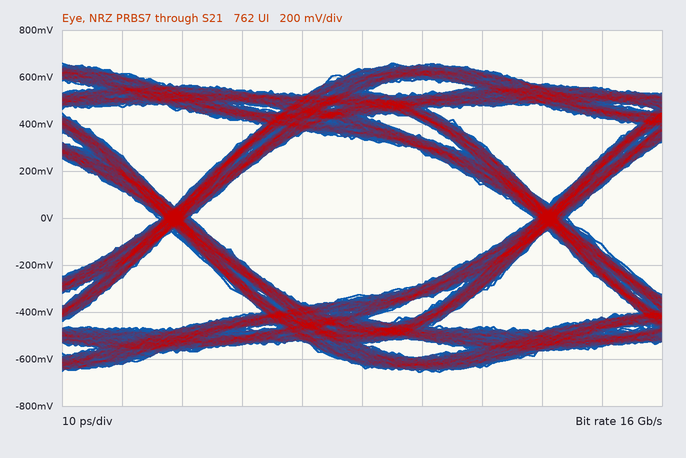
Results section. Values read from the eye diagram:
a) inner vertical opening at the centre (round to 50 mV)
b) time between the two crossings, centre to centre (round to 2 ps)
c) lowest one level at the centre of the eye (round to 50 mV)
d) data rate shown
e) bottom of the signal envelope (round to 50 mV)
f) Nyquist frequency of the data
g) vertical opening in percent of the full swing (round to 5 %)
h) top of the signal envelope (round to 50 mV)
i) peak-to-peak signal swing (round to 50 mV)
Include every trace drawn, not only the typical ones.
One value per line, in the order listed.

650 mV
62 ps
350 mV
16 Gb/s
-650 mV
8 GHz
50 %
650 mV
1.30 V
